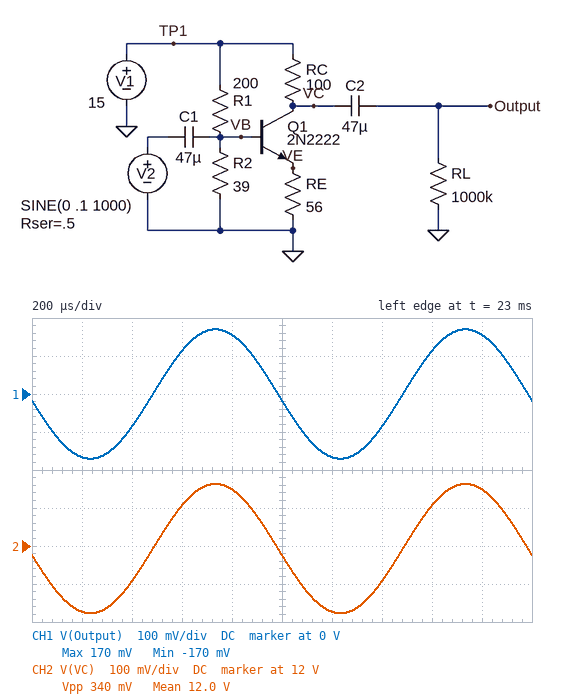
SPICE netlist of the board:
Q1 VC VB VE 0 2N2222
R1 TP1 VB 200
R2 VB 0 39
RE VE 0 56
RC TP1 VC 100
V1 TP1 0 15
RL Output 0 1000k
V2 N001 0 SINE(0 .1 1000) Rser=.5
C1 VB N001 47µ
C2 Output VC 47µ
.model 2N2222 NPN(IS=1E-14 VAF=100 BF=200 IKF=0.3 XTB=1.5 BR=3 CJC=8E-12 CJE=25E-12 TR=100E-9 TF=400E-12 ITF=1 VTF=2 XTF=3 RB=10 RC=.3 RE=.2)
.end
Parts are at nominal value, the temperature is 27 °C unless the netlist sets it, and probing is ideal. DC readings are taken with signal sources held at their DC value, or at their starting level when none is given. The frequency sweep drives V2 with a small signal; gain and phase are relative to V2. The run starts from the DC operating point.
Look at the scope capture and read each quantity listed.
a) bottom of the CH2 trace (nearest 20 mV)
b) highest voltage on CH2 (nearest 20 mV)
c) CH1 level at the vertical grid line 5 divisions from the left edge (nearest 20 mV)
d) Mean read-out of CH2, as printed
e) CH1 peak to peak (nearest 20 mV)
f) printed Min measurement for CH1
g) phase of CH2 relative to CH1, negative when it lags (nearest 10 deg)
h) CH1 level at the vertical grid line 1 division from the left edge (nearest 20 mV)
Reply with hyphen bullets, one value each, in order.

- 11.82 V
- 12.16 V
- -20 mV
- 12.0 V
- 340 mV
- -170 mV
- 0 deg
- -160 mV
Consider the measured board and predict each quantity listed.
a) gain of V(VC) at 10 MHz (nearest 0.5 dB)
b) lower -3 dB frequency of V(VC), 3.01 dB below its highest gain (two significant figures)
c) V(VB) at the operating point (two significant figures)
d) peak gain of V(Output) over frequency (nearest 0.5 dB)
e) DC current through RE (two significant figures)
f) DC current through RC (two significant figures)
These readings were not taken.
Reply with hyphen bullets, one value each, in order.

- 4.5 dB
- 100 Hz
- 2.4 V
- 4.5 dB
- 30 mA
- 30 mA
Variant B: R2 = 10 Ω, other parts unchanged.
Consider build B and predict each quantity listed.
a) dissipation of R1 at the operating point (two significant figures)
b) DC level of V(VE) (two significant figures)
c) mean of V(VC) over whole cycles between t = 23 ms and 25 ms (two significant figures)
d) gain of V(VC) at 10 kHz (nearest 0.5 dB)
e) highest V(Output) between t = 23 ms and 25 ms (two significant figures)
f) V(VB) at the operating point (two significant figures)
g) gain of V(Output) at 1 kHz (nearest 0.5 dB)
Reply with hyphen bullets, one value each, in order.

- 1.0 W
- 60 mV
- 15 V
- 1.5 dB
- 86 mV
- 710 mV
- 1.0 dB
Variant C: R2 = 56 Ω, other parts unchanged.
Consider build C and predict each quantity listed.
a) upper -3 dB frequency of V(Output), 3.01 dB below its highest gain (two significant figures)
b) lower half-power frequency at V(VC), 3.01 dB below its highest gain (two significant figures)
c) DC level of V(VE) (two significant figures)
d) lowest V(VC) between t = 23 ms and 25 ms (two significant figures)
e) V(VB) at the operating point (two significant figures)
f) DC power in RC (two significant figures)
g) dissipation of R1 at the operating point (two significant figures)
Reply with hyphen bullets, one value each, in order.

- 340 MHz
- 77 Hz
- 2.5 V
- 10 V
- 3.3 V
- 200 mW
- 690 mW
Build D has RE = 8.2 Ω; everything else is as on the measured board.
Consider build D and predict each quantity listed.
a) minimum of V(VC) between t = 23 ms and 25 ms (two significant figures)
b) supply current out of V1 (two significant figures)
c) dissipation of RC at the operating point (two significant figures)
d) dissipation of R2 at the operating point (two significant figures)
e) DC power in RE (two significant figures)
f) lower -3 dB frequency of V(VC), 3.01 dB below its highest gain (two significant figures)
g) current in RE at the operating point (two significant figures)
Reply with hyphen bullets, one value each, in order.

- 1.3 V
- 200 mA
- 1.9 W
- 120 mW
- 180 mW
- 150 kHz
- 150 mA
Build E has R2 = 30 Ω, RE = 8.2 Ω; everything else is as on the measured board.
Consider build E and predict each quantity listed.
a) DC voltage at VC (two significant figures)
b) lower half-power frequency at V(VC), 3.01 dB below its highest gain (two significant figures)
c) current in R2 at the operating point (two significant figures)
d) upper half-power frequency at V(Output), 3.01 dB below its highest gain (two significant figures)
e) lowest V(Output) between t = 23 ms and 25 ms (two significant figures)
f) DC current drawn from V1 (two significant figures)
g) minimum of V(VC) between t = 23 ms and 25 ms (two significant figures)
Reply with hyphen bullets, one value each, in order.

- 1.6 V
- 130 Hz
- 64 mA
- 47 MHz
- -330 mV
- 200 mA
- 1.3 V
